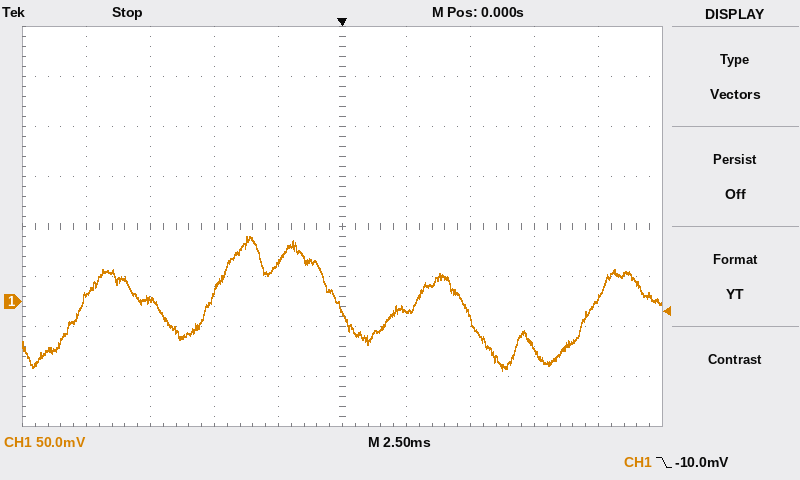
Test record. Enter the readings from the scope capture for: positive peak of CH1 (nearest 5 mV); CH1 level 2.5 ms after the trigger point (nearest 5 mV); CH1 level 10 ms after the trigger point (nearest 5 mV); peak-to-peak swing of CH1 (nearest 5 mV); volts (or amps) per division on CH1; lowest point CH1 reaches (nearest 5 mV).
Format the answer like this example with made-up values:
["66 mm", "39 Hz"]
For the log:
["65 mV", "-10 mV", "5 mV", "135 mV", "50 mV", "-70 mV"]
